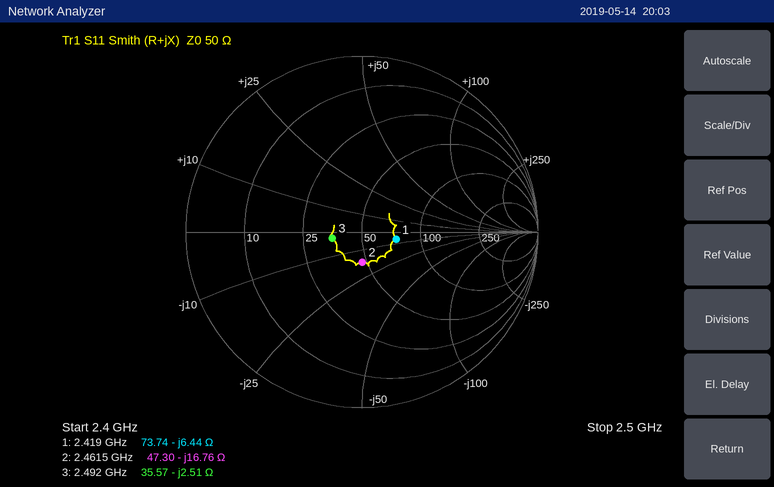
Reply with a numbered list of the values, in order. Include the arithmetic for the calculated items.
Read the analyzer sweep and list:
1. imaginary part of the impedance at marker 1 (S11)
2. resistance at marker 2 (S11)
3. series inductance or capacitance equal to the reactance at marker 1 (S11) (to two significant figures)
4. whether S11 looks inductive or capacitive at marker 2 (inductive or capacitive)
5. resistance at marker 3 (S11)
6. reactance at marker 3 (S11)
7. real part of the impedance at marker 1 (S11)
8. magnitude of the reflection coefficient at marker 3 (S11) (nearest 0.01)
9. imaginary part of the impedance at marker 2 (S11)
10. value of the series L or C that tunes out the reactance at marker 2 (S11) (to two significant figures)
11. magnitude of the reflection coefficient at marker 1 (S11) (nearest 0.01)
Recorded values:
1. -6.44 Ω
2. 47.30 Ω
3. C = 1/(2π × 2.419 GHz × 6.44 Ω) ≈ 10 pF
4. capacitive
5. 35.57 Ω
6. -2.51 Ω
7. 73.74 Ω
8. 0.17
9. -16.76 Ω
10. L = 16.76 Ω/(2π × 2.4615 GHz) ≈ 1.1 nH
11. 0.20
